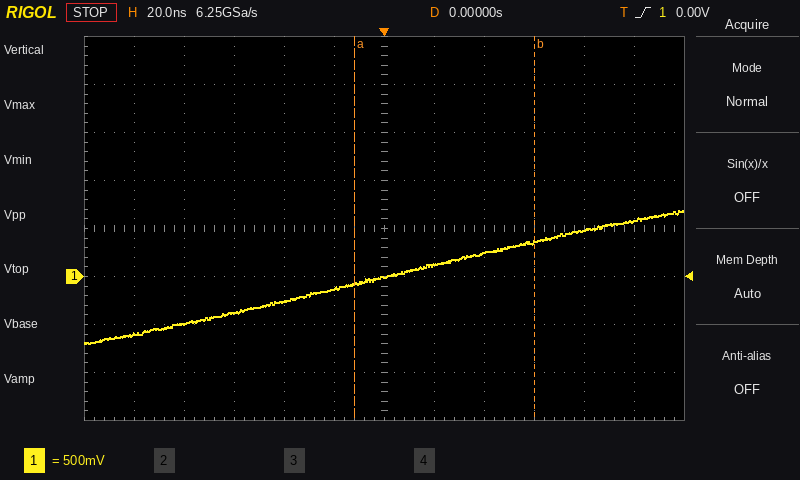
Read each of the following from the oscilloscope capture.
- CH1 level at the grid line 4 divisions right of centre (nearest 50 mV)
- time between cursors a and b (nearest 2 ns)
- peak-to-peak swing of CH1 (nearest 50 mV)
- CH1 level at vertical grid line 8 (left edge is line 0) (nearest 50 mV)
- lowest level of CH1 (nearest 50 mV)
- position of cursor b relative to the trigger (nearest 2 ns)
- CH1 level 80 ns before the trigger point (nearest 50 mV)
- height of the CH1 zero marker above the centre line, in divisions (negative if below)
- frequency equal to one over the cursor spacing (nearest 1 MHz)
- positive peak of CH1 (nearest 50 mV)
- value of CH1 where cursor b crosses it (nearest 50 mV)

500 mV
72 ns
1.40 V
250 mV
-700 mV
+60 ns
-500 mV
-1.0 div
14 MHz
700 mV
350 mV
